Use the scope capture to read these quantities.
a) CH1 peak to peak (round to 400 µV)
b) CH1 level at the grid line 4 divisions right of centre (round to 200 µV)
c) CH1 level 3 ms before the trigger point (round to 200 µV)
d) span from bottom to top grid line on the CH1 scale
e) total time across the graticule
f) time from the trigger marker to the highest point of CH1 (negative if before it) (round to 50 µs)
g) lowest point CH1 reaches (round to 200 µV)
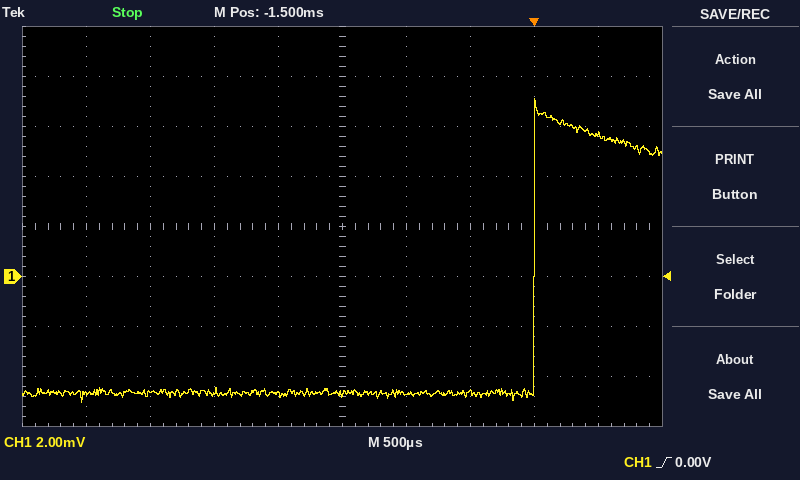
12.0 mV
5.6 mV
-4.6 mV
16 mV
5 ms
0 µs
-5.0 mV
